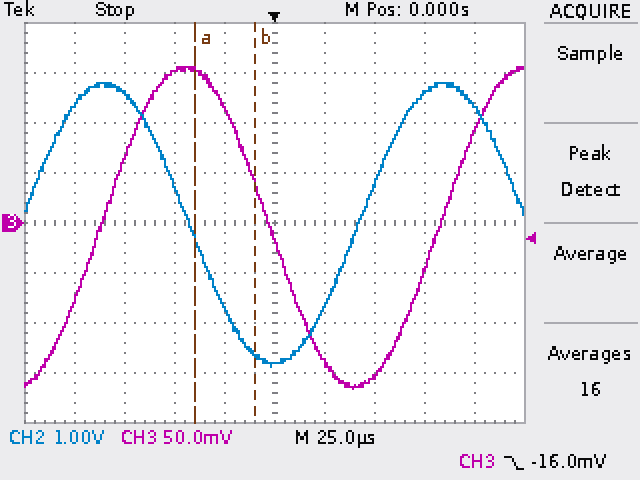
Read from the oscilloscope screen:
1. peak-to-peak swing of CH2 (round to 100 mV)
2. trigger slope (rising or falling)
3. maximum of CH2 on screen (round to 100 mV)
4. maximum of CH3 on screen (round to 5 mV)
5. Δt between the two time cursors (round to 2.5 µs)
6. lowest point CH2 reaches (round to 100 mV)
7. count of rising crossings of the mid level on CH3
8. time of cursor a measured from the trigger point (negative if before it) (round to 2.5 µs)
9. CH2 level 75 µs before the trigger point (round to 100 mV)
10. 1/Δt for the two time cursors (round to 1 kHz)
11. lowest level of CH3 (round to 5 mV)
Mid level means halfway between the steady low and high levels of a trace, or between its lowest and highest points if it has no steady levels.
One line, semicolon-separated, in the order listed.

5.7 V; falling; 2.8 V; 155 mV; 30.0 µs; -2.9 V; 2; -40.0 µs; 2.6 V; 33 kHz; -165 mV
